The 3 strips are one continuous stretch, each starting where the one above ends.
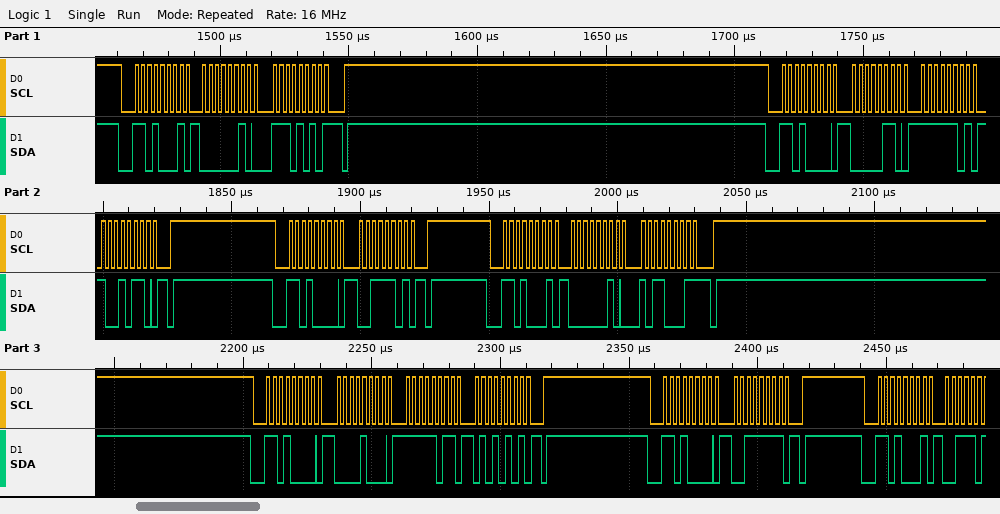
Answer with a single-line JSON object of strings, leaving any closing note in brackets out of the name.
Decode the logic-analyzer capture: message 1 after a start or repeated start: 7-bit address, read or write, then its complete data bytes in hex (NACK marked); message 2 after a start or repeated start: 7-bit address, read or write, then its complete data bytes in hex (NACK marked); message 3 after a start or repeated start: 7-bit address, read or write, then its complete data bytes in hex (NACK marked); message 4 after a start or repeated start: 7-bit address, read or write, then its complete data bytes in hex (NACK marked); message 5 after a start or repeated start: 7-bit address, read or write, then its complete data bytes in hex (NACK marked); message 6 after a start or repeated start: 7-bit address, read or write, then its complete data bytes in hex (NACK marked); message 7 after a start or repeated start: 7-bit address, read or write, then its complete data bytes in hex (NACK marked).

{"message 1 after a start or repeated start: 7-bit address, read or write, then its complete data bytes in hex": "0x68 read: 02 EA NACK", "message 2 after a start or repeated start: 7-bit address, read or write, then its complete data bytes in hex": "0x68 write: 06 FD 96", "message 3 after a start or repeated start: 7-bit address, read or write, then its complete data bytes in hex": "0x68 write: 3D", "message 4 after a start or repeated start: 7-bit address, read or write, then its complete data bytes in hex": "0x68 read: 02 B1 NACK", "message 5 after a start or repeated start: 7-bit address, read or write, then its complete data bytes in hex": "0x68 write: 08 FB 55", "message 6 after a start or repeated start: 7-bit address, read or write, then its complete data bytes in hex": "0x68 write: 3F", "message 7 after a start or repeated start: 7-bit address, read or write, then its complete data bytes in hex": "0x68 read"}
